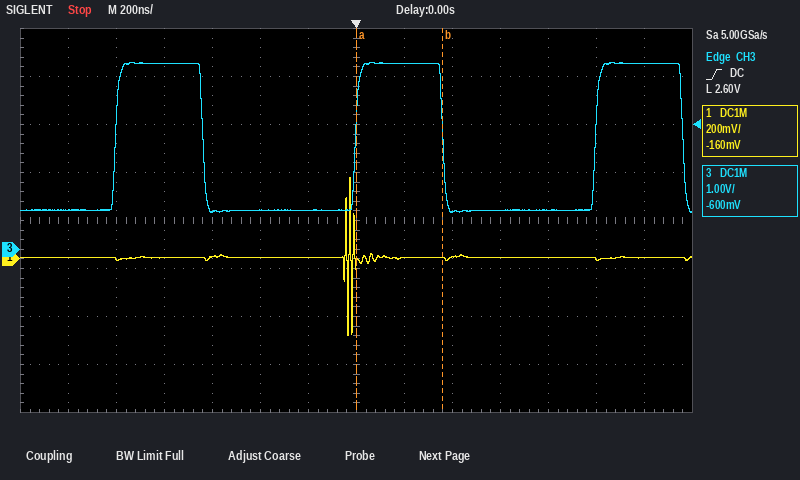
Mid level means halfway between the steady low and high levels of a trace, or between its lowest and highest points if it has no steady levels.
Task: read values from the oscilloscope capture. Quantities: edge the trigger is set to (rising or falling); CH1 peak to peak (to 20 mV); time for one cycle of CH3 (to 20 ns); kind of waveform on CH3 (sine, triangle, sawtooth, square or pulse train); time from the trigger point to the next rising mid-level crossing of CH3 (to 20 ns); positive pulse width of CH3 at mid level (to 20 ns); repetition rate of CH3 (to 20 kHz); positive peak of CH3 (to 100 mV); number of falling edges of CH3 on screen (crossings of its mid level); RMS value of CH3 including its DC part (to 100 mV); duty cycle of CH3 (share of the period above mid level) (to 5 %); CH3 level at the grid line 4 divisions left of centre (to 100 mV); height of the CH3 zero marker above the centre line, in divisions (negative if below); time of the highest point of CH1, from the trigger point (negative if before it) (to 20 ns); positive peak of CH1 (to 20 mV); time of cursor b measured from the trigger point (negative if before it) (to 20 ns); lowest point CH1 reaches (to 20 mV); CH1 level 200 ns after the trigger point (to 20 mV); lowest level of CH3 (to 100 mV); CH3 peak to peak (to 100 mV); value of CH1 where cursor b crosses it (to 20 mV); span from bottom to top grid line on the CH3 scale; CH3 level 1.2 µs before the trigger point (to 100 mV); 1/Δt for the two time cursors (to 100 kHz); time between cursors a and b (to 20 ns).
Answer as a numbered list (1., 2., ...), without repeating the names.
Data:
1. rising
2. 660 mV
3. 1.00 µs
4. pulse train
5. 1.00 µs
6. 360 ns
7. 1.00 MHz
8. 3.9 V
9. 3
10. 2.4 V
11. 35 %
12. 3.9 V
13. -0.6 div
14. -20 ns
15. 340 mV
16. +360 ns
17. -320 mV
18. 0 mV
19. 800 mV
20. 3.1 V
21. 0 mV
22. 8 V
23. 800 mV
24. 2.8 MHz
25. 360 ns
